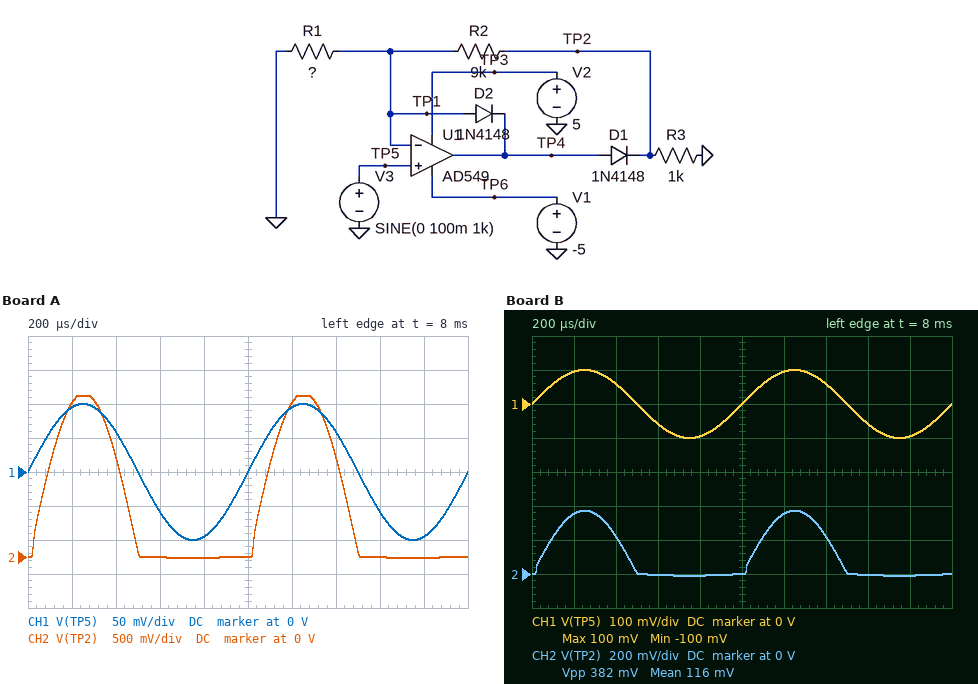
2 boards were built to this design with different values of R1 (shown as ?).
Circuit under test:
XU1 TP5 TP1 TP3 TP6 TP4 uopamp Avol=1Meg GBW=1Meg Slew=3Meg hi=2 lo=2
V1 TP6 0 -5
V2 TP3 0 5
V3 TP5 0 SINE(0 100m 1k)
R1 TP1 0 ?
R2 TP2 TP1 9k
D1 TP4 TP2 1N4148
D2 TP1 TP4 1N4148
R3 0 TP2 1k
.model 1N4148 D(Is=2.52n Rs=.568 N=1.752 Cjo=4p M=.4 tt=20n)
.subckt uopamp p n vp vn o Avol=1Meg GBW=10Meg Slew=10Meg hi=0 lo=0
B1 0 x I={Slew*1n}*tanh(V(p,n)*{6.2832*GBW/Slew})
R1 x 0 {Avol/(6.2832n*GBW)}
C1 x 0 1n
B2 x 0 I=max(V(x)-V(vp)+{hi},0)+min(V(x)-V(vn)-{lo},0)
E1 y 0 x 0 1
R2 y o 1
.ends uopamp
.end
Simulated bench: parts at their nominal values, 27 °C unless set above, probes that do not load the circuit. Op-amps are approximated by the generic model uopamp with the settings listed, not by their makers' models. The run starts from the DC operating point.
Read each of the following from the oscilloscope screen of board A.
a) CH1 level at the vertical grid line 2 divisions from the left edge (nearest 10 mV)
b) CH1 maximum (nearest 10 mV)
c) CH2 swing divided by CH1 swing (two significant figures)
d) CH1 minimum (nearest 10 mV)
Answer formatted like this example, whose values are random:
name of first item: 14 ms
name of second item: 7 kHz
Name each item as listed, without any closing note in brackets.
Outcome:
CH1 level at the vertical grid line 2 divisions from the left edge: 60 mV
CH1 maximum: 100 mV
CH2 swing divided by CH1 swing: 12
CH1 minimum: -100 mV
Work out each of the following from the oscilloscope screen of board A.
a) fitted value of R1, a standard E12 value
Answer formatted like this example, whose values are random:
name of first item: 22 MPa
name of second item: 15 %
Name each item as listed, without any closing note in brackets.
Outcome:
fitted value of R1, a standard E12 value: 390 Ω
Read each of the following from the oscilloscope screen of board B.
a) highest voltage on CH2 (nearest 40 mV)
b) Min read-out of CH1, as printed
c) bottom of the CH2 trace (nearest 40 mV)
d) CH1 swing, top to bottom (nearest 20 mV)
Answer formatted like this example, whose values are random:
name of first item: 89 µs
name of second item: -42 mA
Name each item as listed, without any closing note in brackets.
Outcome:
highest voltage on CH2: 360 mV
Min read-out of CH1, as printed: -100 mV
bottom of the CH2 trace: 0 V
CH1 swing, top to bottom: 200 mV
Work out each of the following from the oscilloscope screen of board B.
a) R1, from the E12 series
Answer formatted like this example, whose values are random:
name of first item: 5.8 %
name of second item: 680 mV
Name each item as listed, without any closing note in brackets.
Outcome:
R1, from the E12 series: 3.3 kΩ
